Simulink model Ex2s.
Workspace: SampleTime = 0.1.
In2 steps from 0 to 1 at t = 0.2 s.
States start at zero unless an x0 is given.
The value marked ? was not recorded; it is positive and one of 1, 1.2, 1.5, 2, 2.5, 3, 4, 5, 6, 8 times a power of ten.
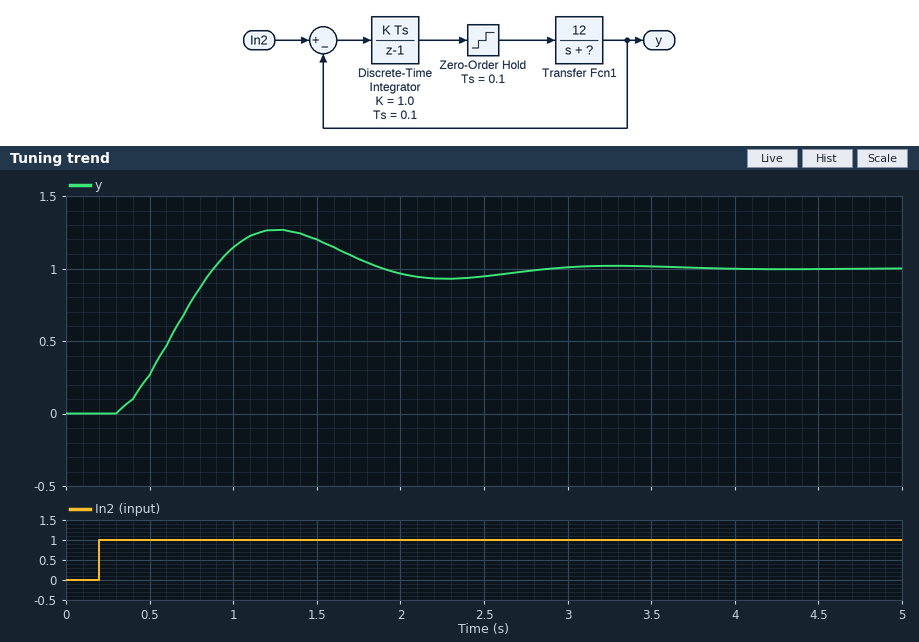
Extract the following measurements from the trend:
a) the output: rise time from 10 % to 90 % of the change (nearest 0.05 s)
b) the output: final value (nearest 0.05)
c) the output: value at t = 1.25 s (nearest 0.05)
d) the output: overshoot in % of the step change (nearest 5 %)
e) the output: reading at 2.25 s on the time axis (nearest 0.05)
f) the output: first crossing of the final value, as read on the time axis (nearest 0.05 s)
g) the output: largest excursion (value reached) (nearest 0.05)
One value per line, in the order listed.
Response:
0.40 s
1.00
1.25
25 %
0.95
0.90 s
1.25
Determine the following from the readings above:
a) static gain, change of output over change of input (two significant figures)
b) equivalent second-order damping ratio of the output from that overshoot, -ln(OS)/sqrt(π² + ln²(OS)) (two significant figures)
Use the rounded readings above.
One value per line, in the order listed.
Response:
1.0
0.40
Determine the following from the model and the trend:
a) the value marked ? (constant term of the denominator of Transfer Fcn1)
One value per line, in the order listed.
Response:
4
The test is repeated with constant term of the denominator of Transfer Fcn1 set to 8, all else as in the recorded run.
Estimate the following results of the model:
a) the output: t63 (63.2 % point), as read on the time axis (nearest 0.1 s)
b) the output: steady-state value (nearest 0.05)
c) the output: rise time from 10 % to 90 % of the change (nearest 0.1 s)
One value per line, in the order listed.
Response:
0.9 s
1.00
0.9 s
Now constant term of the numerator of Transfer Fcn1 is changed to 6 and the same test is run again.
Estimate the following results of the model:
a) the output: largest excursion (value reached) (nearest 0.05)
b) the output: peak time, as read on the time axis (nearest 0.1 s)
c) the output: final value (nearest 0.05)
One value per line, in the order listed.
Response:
1.05
2.0 s
1.00
